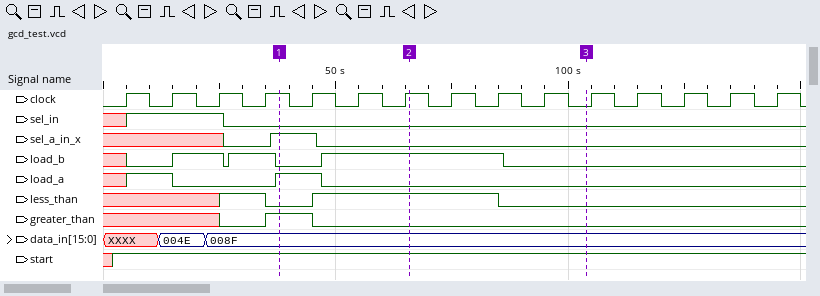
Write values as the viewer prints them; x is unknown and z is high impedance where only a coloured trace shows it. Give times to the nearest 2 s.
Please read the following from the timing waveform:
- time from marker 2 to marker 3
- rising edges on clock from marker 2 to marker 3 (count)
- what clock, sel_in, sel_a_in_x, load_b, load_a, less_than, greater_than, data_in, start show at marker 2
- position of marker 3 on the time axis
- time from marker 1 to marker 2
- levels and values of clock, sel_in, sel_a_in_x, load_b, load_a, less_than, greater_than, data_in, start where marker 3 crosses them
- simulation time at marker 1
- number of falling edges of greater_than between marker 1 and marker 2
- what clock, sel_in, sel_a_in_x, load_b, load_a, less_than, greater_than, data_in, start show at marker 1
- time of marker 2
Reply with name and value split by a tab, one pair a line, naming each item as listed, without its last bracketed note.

time from marker 2 to marker 3	38 s
rising edges on clock from marker 2 to marker 3	3
what clock, sel_in, sel_a_in_x, load_b, load_a, less_than, greater_than, data_in, start show at marker 2	clock=1, sel_in=0, sel_a_in_x=0, load_b=1, load_a=0, less_than=1, greater_than=0, data_in=008F, start=1
position of marker 3 on the time axis	104 s
time from marker 1 to marker 2	28 s
levels and values of clock, sel_in, sel_a_in_x, load_b, load_a, less_than, greater_than, data_in, start where marker 3 crosses them	clock=0, sel_in=0, sel_a_in_x=0, load_b=0, load_a=0, less_than=0, greater_than=0, data_in=008F, start=1
simulation time at marker 1	38 s
number of falling edges of greater_than between marker 1 and marker 2	1
what clock, sel_in, sel_a_in_x, load_b, load_a, less_than, greater_than, data_in, start show at marker 1	clock=1, sel_in=0, sel_a_in_x=1, load_b=0, load_a=1, less_than=0, greater_than=1, data_in=008F, start=1
time of marker 2	66 s
